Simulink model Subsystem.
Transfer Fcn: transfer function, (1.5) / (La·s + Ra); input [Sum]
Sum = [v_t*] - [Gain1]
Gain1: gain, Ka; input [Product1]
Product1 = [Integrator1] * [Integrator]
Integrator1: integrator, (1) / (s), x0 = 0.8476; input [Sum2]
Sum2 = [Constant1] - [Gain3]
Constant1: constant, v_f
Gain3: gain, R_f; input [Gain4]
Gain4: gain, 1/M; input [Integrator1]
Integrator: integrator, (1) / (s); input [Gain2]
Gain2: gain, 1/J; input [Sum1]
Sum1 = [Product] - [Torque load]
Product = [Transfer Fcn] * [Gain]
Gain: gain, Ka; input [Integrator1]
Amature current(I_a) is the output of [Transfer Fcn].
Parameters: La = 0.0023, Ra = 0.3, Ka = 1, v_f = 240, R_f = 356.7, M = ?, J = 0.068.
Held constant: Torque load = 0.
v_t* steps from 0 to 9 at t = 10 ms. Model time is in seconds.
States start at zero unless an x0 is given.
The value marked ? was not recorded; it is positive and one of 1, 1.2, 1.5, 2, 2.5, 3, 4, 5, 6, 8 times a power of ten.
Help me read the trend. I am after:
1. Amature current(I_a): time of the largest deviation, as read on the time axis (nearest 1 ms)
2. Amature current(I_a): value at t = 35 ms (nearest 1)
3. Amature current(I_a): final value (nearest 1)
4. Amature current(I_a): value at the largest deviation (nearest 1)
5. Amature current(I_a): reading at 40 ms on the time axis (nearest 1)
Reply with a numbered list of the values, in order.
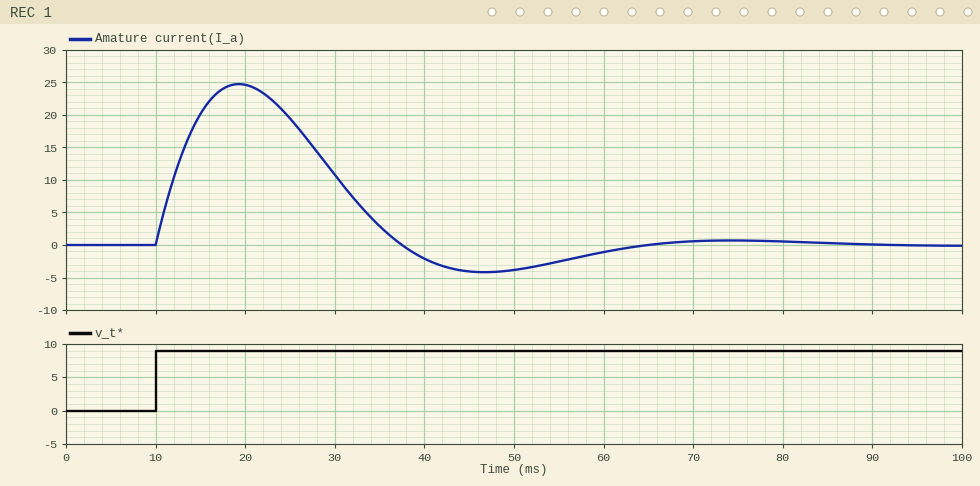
1. 19 ms
2. 3
3. 0
4. 25
5. -2
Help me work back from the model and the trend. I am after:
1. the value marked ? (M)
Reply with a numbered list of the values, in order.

1. 2
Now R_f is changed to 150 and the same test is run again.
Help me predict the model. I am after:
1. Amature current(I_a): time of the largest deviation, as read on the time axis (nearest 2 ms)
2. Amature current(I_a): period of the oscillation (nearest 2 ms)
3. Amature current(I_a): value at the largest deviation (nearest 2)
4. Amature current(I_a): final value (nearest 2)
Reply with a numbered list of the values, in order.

1. 16 ms
2. 24 ms
3. 18
4. 0
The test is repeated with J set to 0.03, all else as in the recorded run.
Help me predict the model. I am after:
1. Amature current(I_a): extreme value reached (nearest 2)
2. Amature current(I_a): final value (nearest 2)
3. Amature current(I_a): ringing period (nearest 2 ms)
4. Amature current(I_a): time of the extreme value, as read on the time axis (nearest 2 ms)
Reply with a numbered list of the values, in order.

1. 20
2. 0
3. 34 ms
4. 16 ms
